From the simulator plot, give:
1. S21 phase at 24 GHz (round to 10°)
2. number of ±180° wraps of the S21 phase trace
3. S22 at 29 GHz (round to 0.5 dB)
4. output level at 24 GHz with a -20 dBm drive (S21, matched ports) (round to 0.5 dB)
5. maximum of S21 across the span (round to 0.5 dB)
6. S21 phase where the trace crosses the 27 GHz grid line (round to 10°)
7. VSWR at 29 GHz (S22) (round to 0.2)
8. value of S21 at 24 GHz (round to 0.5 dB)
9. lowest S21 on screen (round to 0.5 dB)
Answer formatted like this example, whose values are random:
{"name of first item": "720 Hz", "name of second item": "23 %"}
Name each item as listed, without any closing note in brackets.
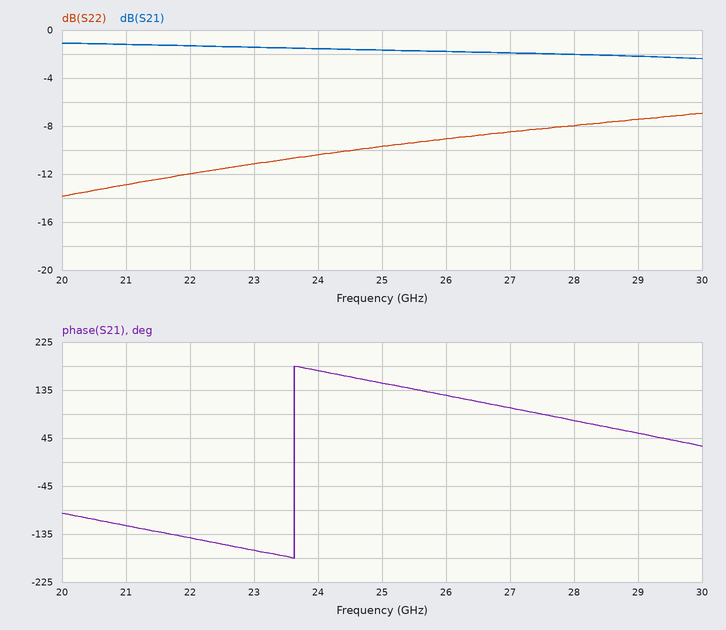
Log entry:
{"S21 phase at 24 GHz": "170°", "number of ±180° wraps of the S21 phase trace": "1", "S22 at 29 GHz": "-7.5 dB", "output level at 24 GHz with a -20 dBm drive (S21, matched ports)": "-21.5 dBm", "maximum of S21 across the span": "-1.0 dB", "S21 phase where the trace crosses the 27 GHz grid line": "100°", "VSWR at 29 GHz (S22)": "2.4", "value of S21 at 24 GHz": "-1.5 dB", "lowest S21 on screen": "-2.5 dB"}
